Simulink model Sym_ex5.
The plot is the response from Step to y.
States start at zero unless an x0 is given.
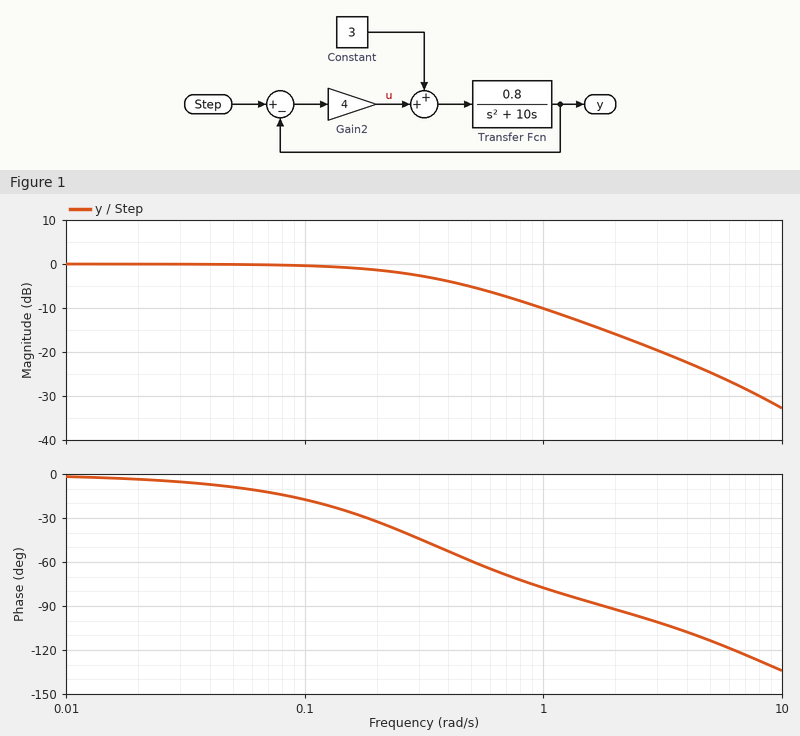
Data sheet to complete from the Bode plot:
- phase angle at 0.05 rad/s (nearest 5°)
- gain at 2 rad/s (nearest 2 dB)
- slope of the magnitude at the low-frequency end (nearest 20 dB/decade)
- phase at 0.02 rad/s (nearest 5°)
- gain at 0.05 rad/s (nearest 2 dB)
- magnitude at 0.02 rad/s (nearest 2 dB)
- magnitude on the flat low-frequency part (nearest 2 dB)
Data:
-10°
-16 dB
0 dB/decade
-5°
0 dB
0 dB
0 dB
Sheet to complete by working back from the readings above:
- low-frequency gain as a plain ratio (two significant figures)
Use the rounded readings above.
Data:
1.0
